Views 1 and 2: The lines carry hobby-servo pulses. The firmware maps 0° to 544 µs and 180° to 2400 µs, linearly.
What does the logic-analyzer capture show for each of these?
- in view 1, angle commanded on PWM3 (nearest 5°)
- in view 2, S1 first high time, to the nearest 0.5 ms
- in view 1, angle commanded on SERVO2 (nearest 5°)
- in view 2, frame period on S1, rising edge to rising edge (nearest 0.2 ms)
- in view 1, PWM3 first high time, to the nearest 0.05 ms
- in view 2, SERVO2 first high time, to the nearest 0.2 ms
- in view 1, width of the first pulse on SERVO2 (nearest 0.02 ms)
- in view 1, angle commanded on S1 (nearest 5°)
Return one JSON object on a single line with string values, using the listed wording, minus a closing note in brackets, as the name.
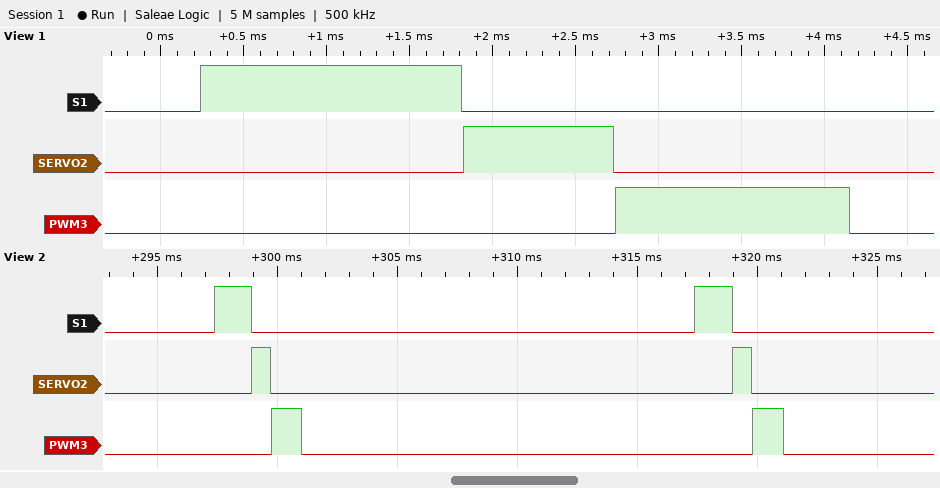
{"in view 1, angle commanded on PWM3": "85°", "in view 2, S1 first high time, to the nearest 0.5 ms": "1.5 ms", "in view 1, angle commanded on SERVO2": "35°", "in view 2, frame period on S1, rising edge to rising edge": "20.0 ms", "in view 1, PWM3 first high time, to the nearest 0.05 ms": "1.40 ms", "in view 2, SERVO2 first high time, to the nearest 0.2 ms": "0.8 ms", "in view 1, width of the first pulse on SERVO2": "0.90 ms", "in view 1, angle commanded on S1": "100°"}
